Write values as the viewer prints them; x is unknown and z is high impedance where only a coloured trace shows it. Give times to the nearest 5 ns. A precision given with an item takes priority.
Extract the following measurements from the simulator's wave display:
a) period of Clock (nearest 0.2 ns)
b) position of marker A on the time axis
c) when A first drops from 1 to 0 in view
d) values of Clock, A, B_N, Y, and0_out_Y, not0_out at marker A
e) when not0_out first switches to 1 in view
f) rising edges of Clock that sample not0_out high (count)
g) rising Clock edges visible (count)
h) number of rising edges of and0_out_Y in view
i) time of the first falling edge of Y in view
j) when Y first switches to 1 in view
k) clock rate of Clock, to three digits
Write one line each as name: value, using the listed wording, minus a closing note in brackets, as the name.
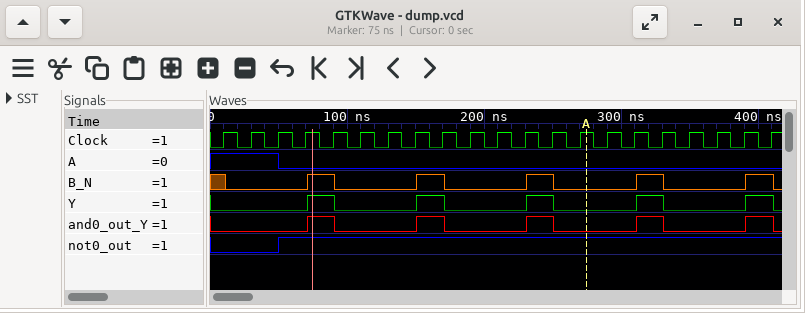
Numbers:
period of Clock: 20 ns
position of marker A on the time axis: 275 ns
when A first drops from 1 to 0 in view: 50 ns
values of Clock, A, B_N, Y, and0_out_Y, not0_out at marker A: Clock=1, A=0, B_N=0, Y=0, and0_out_Y=0, not0_out=1
when not0_out first switches to 1 in view: 50 ns
rising edges of Clock that sample not0_out high: 18
rising Clock edges visible: 21
number of rising edges of and0_out_Y in view: 5
time of the first falling edge of Y in view: 90 ns
when Y first switches to 1 in view: 70 ns
clock rate of Clock, to three digits: 50.0 MHz
